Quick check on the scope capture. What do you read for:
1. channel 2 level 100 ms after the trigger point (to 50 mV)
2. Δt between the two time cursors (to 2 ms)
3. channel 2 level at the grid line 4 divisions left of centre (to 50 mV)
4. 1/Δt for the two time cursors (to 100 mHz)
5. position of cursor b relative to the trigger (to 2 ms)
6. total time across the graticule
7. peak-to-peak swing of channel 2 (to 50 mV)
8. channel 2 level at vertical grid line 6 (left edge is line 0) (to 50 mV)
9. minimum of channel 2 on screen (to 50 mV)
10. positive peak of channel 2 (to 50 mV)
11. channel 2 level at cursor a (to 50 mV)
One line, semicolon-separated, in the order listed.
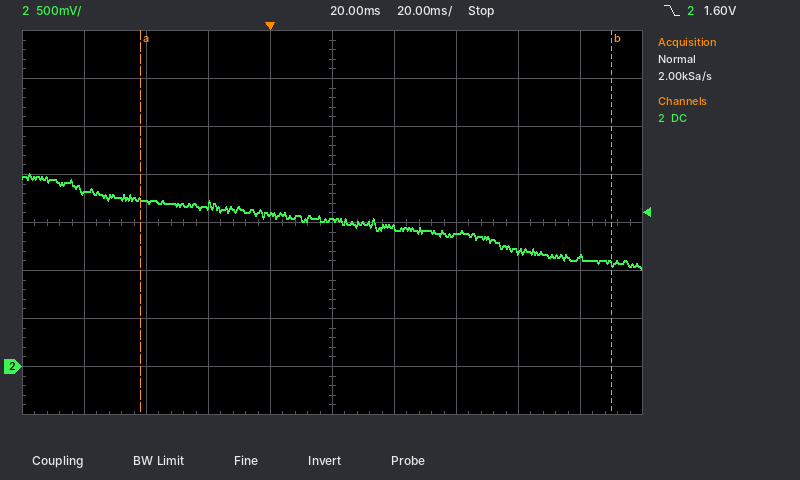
1.15 V; 152 ms; 1.80 V; 6.6 Hz; +110 ms; 200 ms; 1.00 V; 1.45 V; 1.00 V; 2.00 V; 1.75 V
